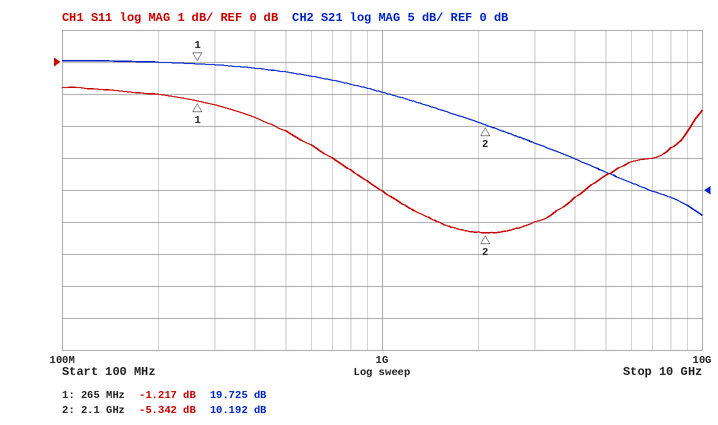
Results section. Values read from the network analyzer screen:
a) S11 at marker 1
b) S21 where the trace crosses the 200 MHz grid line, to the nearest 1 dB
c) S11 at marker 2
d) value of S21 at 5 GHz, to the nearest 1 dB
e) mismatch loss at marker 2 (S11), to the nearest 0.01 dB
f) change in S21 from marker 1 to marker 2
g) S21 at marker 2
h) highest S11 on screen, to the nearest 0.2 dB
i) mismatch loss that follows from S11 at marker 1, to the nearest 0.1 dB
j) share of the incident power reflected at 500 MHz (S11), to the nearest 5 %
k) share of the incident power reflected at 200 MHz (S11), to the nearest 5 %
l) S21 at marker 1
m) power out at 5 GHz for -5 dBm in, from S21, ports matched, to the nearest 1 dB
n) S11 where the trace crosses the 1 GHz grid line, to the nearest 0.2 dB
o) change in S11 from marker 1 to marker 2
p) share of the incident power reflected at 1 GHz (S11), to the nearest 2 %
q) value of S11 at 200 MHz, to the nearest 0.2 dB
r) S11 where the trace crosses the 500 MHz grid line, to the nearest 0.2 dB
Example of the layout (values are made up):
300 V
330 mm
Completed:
-1.217 dB
20 dB
-5.342 dB
3 dB
1.50 dB
-9.533 dB
10.192 dB
-0.8 dB
6.1 dB
60 %
80 %
19.725 dB
-2 dBm
-4.0 dB
-4.125 dB
40 %
-1.0 dB
-2.2 dB
